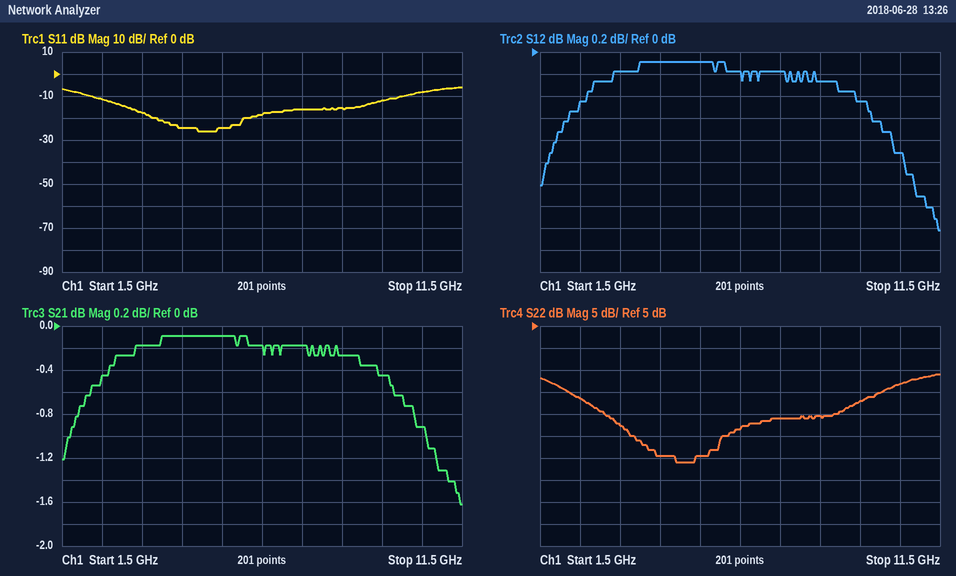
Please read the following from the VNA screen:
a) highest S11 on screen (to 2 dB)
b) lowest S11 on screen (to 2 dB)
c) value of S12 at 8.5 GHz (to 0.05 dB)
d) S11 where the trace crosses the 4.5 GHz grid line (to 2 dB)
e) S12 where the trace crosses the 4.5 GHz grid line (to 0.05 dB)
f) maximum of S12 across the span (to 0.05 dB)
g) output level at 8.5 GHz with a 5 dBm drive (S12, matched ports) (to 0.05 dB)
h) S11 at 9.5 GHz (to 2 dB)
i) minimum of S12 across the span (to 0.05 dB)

-6 dB
-26 dB
-0.25 dB
-24 dB
-0.10 dB
-0.10 dB
4.75 dBm
-12 dB
-1.60 dB
